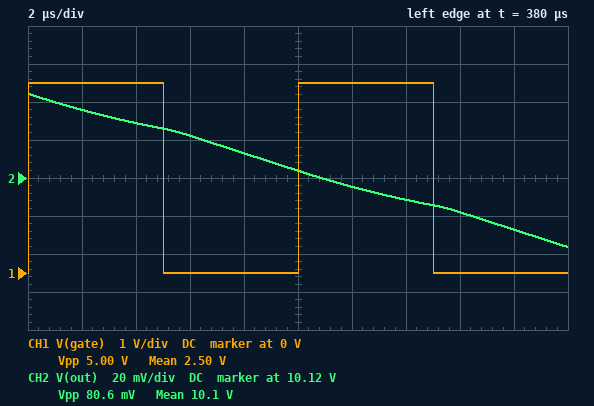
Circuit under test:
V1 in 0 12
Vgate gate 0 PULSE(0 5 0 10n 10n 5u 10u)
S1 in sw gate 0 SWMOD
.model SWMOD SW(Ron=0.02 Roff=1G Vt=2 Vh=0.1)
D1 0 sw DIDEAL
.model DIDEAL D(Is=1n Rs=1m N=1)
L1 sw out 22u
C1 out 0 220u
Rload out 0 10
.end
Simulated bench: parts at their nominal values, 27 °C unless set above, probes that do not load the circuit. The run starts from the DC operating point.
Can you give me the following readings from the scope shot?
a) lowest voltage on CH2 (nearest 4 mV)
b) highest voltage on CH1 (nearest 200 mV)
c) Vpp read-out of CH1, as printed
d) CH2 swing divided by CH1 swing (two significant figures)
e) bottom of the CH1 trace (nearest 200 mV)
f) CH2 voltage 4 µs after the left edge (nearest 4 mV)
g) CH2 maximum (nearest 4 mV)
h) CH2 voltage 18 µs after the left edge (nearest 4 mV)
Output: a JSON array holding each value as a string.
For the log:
["10.084 V", "5.0 V", "5.00 V", "0.016", "0 V", "10.148 V", "10.164 V", "10.092 V"]
